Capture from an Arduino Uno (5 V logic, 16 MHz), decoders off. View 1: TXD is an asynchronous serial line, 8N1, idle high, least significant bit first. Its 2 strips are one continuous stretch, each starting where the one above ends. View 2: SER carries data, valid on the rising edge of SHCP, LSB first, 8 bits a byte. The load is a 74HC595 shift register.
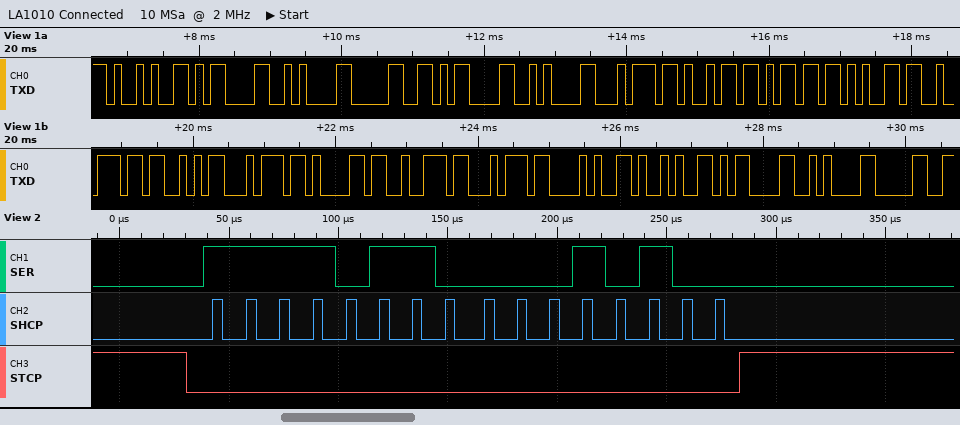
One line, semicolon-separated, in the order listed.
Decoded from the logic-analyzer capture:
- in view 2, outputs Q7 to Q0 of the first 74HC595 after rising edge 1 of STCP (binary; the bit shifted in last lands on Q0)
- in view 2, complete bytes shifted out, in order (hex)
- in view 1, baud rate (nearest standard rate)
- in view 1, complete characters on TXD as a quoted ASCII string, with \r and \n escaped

00010100; 6F 28; 9600 baud; ")\r\n0\r\ntimerStart()\r\n0"
